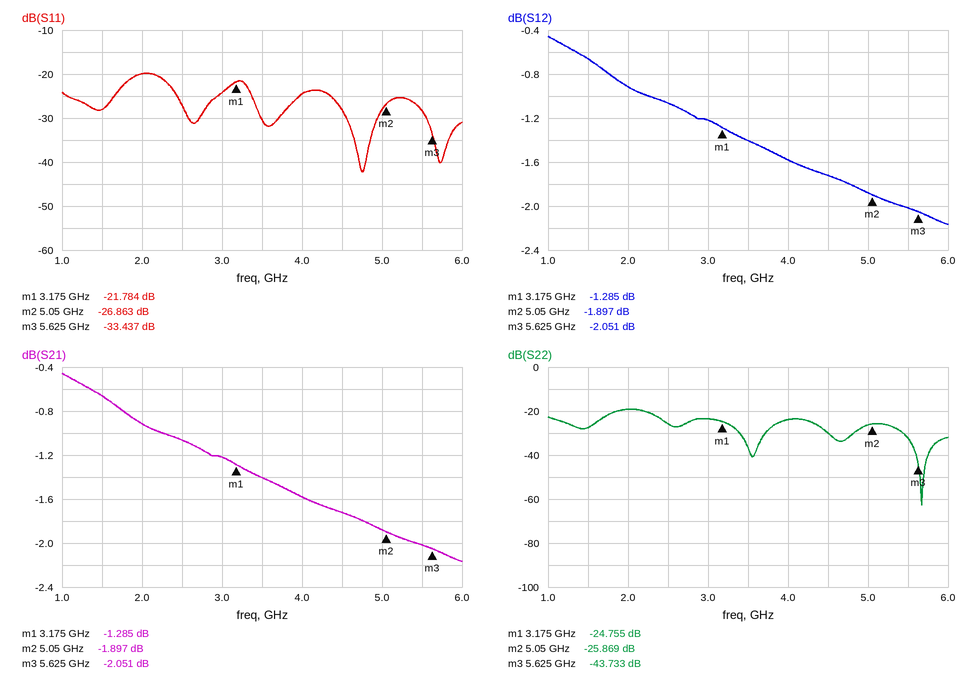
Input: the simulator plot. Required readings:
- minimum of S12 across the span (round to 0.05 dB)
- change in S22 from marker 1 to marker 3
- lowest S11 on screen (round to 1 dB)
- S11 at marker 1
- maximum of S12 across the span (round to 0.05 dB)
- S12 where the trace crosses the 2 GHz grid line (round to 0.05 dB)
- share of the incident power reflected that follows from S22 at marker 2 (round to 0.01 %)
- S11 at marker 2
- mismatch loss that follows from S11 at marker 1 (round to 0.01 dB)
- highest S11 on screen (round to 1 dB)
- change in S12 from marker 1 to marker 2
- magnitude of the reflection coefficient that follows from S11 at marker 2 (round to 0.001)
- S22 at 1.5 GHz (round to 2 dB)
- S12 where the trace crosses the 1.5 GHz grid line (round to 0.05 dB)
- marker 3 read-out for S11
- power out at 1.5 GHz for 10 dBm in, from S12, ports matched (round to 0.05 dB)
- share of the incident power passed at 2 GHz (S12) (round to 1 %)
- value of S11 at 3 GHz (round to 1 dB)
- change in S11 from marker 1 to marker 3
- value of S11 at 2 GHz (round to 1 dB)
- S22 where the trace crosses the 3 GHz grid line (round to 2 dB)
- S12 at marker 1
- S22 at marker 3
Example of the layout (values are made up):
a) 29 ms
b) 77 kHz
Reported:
a) -2.15 dB
b) -18.978 dB
c) -42 dB
d) -21.784 dB
e) -0.45 dB
f) -0.90 dB
g) 0.26 %
h) -26.863 dB
i) 0.03 dB
j) -20 dB
k) -0.612 dB
l) 0.045
m) -28 dB
n) -0.65 dB
o) -33.437 dB
p) 9.35 dBm
q) 81 %
r) -24 dB
s) -11.653 dB
t) -20 dB
u) -24 dB
v) -1.285 dB
w) -43.733 dB
